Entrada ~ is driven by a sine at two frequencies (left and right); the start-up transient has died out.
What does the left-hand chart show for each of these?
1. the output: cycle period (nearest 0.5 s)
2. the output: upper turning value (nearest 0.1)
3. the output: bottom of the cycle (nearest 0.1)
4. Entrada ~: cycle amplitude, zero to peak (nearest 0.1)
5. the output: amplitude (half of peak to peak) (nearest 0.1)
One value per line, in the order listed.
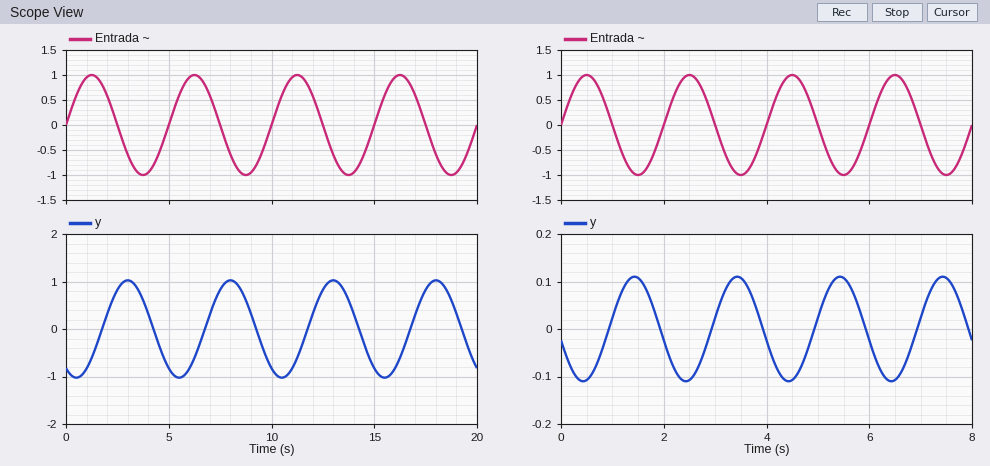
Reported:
5.0 s
1.0
-1.0
1.0
1.0
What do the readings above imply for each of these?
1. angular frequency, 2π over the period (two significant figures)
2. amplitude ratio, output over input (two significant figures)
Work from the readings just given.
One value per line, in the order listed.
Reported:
1.3 rad/s
1.0
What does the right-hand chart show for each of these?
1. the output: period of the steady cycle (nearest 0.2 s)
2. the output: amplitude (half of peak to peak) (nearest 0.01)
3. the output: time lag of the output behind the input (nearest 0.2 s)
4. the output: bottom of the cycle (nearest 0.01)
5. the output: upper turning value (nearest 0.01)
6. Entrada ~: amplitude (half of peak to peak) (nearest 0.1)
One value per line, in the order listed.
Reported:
2.0 s
0.11
1.0 s
-0.11
0.11
1.0
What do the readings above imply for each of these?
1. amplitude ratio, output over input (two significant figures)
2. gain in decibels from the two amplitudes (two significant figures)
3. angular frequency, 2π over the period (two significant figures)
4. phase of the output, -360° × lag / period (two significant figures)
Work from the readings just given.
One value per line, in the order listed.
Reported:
0.11
-19 dB
3.1 rad/s
-180°
